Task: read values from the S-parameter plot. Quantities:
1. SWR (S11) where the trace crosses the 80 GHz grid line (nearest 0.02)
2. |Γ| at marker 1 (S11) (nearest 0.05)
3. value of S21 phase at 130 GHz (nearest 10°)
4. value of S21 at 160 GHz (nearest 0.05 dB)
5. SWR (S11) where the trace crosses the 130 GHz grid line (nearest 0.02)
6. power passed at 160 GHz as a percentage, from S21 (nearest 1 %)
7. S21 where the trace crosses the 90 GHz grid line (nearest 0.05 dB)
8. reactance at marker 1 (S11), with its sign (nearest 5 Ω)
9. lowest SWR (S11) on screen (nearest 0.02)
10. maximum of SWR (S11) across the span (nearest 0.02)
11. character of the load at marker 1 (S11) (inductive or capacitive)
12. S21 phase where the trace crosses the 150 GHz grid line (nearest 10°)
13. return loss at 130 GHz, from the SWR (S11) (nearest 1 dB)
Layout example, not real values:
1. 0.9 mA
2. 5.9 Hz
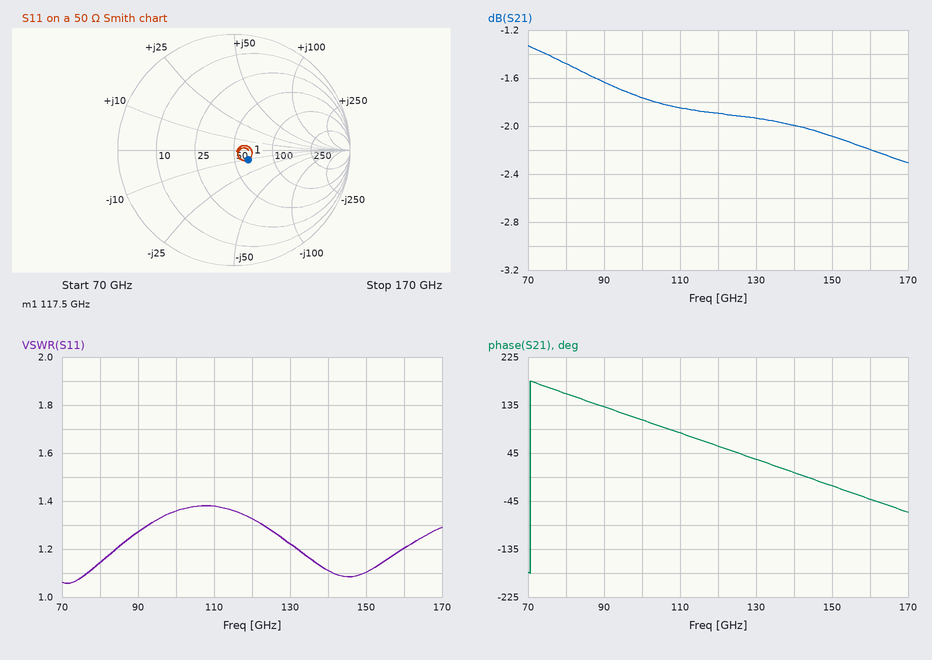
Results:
1. 1.14
2. 0.15
3. 30°
4. -2.20 dB
5. 1.22
6. 60 %
7. -1.65 dB
8. -10 Ω
9. 1.06
10. 1.38
11. capacitive
12. -20°
13. 20 dB
